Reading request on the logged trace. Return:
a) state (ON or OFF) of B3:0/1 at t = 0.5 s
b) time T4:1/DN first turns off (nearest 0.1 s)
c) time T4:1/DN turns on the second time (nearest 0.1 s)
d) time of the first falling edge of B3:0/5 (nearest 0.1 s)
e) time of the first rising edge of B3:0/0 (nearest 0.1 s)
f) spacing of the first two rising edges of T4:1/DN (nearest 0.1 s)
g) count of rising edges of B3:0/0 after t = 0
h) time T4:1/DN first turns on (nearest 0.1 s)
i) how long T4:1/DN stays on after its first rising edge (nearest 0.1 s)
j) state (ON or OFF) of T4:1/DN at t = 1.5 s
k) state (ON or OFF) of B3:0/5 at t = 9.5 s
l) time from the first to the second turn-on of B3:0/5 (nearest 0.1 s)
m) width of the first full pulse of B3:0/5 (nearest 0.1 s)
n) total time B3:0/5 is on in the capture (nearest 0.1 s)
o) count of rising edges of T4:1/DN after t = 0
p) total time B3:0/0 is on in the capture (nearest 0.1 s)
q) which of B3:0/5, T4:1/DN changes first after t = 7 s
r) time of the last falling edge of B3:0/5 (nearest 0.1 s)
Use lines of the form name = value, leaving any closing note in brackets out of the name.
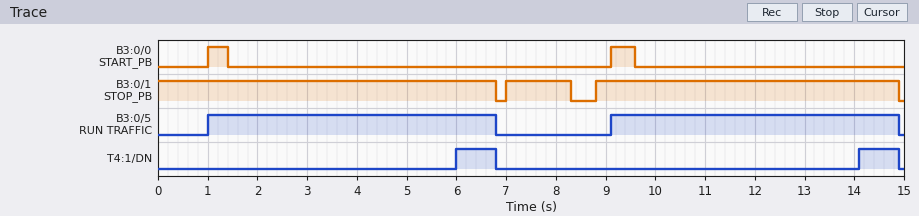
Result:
state (ON or OFF) of B3:0/1 at t = 0.5 s = ON
time T4:1/DN first turns off = 6.8 s
time T4:1/DN turns on the second time = 14.1 s
time of the first falling edge of B3:0/5 = 6.8 s
time of the first rising edge of B3:0/0 = 1.0 s
spacing of the first two rising edges of T4:1/DN = 8.1 s
count of rising edges of B3:0/0 after t = 0 = 2
time T4:1/DN first turns on = 6.0 s
how long T4:1/DN stays on after its first rising edge = 0.8 s
state (ON or OFF) of T4:1/DN at t = 1.5 s = OFF
state (ON or OFF) of B3:0/5 at t = 9.5 s = ON
time from the first to the second turn-on of B3:0/5 = 8.1 s
width of the first full pulse of B3:0/5 = 5.8 s
total time B3:0/5 is on in the capture = 11.6 s
count of rising edges of T4:1/DN after t = 0 = 2
total time B3:0/0 is on in the capture = 0.9 s
which of B3:0/5, T4:1/DN changes first after t = 7 s = B3:0/5
time of the last falling edge of B3:0/5 = 14.9 s
